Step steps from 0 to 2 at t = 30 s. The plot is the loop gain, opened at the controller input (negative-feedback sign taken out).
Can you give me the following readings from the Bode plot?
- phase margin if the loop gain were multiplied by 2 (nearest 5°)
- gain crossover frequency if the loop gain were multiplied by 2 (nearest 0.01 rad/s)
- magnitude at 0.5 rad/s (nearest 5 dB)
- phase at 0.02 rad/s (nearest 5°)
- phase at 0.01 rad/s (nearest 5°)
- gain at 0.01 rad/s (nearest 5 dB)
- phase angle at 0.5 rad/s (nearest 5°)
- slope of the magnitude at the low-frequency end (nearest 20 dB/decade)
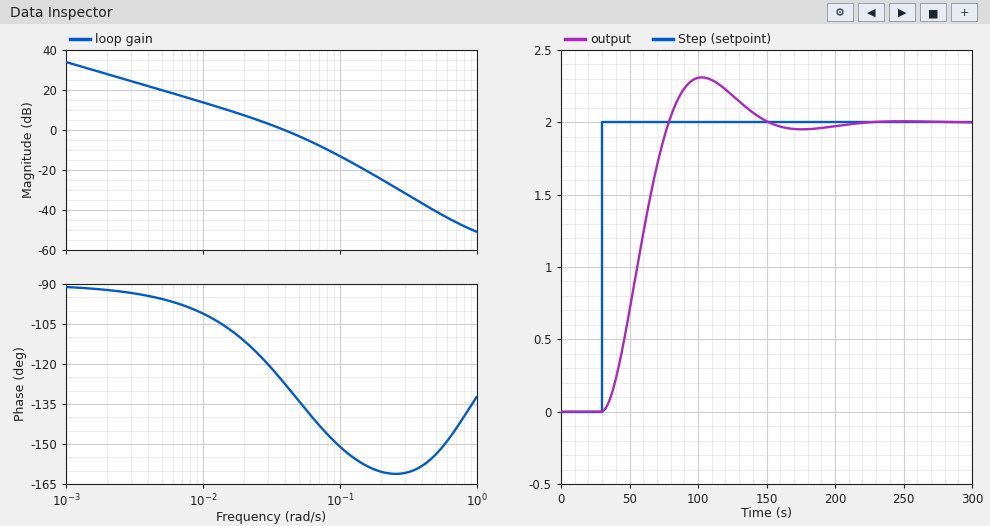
40°
0.06 rad/s
-40 dB
-110°
-100°
15 dB
-155°
-20 dB/decade
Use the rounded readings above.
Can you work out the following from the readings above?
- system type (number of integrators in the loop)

1
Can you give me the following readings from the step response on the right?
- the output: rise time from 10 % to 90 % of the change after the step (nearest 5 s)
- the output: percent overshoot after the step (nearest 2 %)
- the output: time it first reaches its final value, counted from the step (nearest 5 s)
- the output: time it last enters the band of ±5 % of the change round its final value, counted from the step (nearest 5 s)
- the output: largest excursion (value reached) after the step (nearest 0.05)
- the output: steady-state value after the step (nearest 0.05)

35 s
16 %
50 s
105 s
2.30
2.00
